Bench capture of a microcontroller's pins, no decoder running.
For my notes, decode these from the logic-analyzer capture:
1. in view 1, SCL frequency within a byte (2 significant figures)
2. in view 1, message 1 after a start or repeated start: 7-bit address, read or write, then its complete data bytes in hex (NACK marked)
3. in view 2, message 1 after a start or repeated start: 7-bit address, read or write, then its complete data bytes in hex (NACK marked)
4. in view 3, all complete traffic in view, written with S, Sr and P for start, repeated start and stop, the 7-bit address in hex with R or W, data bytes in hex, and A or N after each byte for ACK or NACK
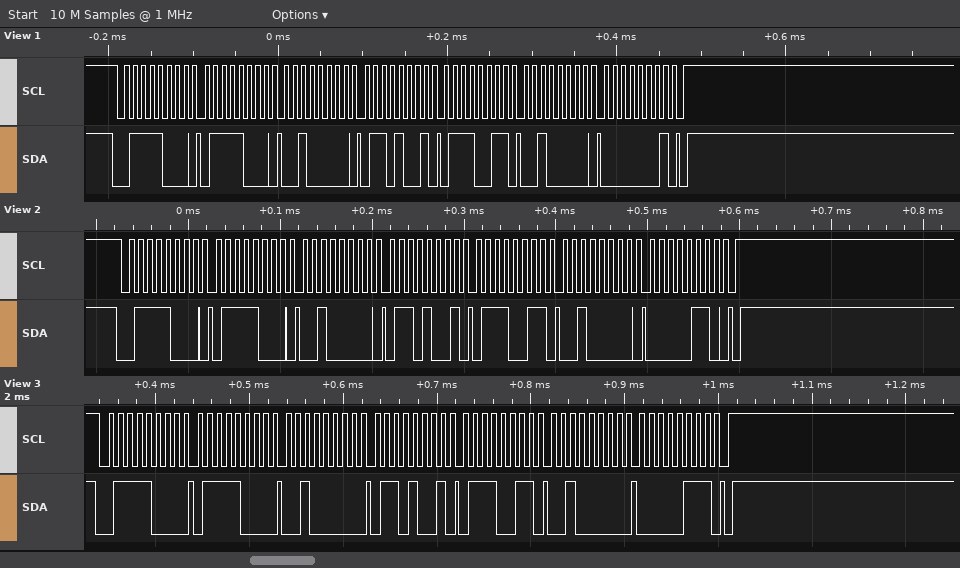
100 kHz
0x3C write: 78 20 69 73 20 01
0x3C write: 78 20 69 73 20 06
S 3CW A 78 A 20 A 69 A 73 A 20 A 07 A P
